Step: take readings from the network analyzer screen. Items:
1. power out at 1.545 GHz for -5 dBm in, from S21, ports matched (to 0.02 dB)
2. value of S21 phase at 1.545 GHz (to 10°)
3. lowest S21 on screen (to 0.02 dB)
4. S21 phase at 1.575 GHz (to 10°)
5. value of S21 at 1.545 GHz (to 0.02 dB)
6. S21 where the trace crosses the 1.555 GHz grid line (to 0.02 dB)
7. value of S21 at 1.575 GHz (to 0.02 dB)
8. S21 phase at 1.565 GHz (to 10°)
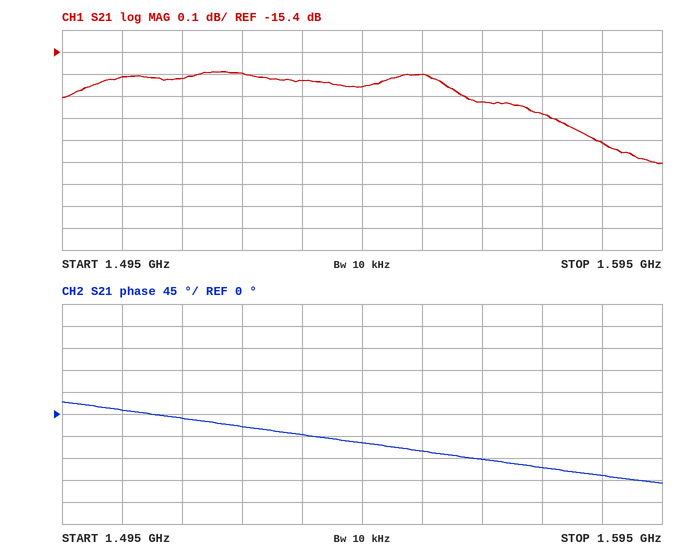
-20.56 dBm
-60°
-15.90 dB
-110°
-15.56 dB
-15.50 dB
-15.68 dB
-90°
